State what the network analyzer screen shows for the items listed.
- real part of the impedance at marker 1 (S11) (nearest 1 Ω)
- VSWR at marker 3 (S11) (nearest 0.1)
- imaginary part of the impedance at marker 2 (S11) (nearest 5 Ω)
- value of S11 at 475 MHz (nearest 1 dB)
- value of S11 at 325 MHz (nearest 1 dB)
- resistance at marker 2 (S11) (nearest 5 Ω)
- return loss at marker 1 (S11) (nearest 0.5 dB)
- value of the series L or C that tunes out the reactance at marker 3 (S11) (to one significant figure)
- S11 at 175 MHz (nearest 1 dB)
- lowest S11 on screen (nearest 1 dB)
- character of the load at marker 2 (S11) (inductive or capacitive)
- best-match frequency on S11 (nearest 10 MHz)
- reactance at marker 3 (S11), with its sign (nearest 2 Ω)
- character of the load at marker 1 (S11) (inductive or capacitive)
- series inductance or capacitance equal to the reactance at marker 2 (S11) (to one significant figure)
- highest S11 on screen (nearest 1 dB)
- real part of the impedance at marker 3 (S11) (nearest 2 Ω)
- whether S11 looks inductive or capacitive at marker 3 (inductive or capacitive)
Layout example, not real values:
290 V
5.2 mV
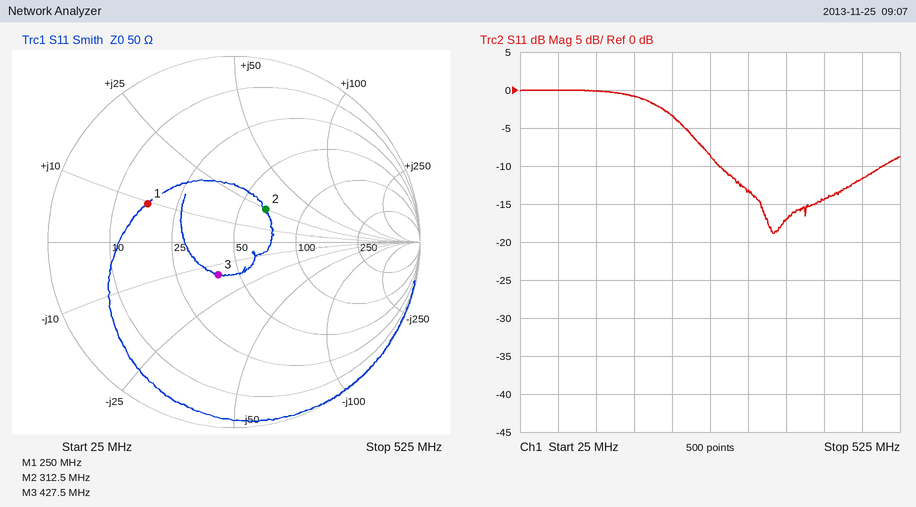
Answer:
17 Ω
1.5
+25 Ω
-12 dB
-13 dB
65 Ω
6.0 dB
5 nH
-1 dB
-19 dB
inductive
360 MHz
-14 Ω
inductive
10 nH
0 dB
40 Ω
capacitive
